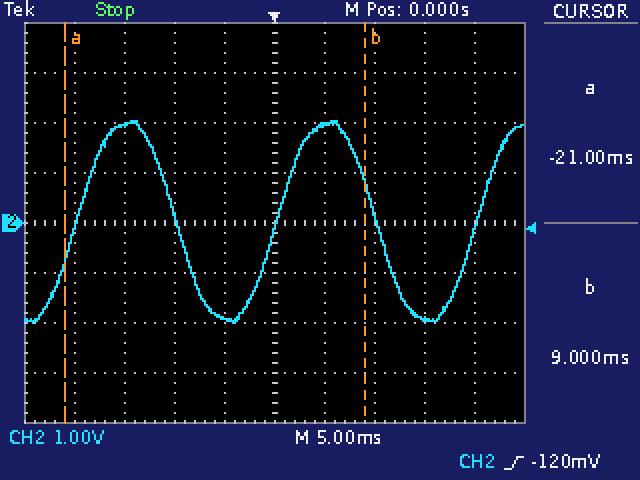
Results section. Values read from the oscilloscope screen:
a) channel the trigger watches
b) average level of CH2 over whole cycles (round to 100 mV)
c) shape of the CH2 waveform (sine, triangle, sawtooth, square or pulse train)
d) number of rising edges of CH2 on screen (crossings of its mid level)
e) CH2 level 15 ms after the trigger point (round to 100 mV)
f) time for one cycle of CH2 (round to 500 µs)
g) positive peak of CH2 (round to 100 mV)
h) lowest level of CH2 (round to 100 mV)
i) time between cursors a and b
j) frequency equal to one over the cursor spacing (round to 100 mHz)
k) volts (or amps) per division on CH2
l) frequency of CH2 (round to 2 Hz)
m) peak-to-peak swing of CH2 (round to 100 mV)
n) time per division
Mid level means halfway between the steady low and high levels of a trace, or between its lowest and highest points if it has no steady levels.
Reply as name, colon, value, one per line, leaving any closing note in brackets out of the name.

channel the trigger watches: CH2
average level of CH2 over whole cycles: 0.0 V
shape of the CH2 waveform: sine
number of rising edges of CH2 on screen: 3
CH2 level 15 ms after the trigger point: -1.9 V
time for one cycle of CH2: 20.0 ms
positive peak of CH2: 2.0 V
lowest level of CH2: -2.0 V
time between cursors a and b: 30.0 ms
frequency equal to one over the cursor spacing: 33.3 Hz
volts (or amps) per division on CH2: 1 V
frequency of CH2: 50 Hz
peak-to-peak swing of CH2: 4.0 V
time per division: 5 ms
